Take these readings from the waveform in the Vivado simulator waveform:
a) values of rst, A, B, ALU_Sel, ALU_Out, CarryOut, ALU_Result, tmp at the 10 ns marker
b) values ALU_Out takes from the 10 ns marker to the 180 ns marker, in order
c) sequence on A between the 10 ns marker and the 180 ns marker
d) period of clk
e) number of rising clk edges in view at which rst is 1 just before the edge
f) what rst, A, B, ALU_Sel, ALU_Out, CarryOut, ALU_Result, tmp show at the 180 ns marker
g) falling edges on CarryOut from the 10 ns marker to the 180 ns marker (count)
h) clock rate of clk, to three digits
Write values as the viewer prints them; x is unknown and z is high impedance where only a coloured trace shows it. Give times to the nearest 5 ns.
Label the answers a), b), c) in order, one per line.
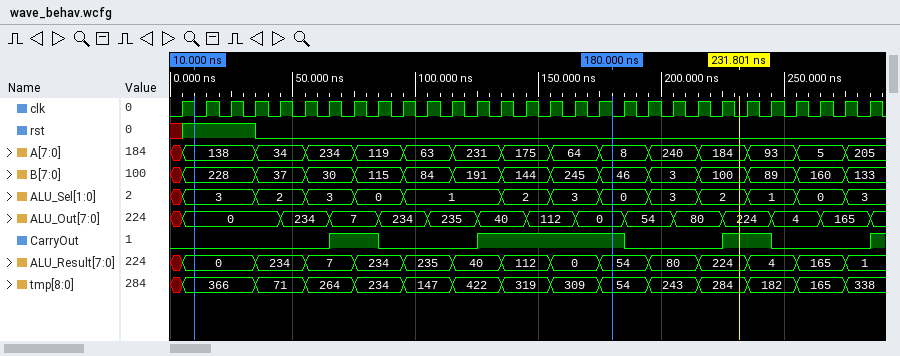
a) rst=1, A=138, B=228, ALU_Sel=3, ALU_Out=0, CarryOut=0, ALU_Result=0, tmp=366
b) 0, 234, 7, 234, 235, 40, 112, 0
c) 138, 34, 234, 119, 63, 231, 175, 64, 8
d) 10 ns
e) 3
f) rst=0, A=8, B=46, ALU_Sel=0, ALU_Out=0, CarryOut=1, ALU_Result=54, tmp=54
g) 1
h) 100 MHz
